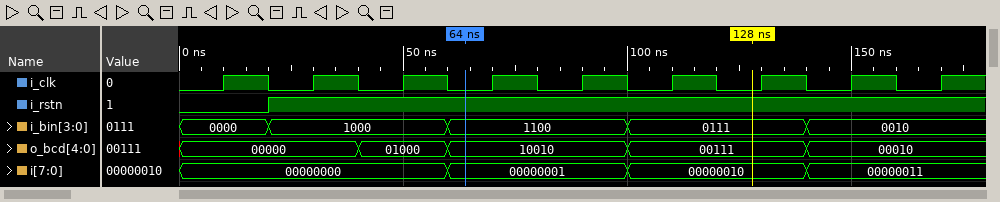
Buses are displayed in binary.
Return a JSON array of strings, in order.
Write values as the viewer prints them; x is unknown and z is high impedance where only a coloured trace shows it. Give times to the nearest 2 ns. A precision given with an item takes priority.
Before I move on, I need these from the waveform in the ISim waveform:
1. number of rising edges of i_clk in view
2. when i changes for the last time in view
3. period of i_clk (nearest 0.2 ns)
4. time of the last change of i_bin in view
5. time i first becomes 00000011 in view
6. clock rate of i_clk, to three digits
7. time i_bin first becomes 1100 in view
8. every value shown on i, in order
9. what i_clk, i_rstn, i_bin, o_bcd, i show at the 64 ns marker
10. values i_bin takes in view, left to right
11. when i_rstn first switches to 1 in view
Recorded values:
["9", "140 ns", "20 ns", "140 ns", "140 ns", "50.0 MHz", "60 ns", "00000000, 00000001, 00000010, 00000011", "i_clk=0, i_rstn=1, i_bin=1100, o_bcd=10010, i=00000001", "0000, 1000, 1100, 0111, 0010", "20 ns"]
